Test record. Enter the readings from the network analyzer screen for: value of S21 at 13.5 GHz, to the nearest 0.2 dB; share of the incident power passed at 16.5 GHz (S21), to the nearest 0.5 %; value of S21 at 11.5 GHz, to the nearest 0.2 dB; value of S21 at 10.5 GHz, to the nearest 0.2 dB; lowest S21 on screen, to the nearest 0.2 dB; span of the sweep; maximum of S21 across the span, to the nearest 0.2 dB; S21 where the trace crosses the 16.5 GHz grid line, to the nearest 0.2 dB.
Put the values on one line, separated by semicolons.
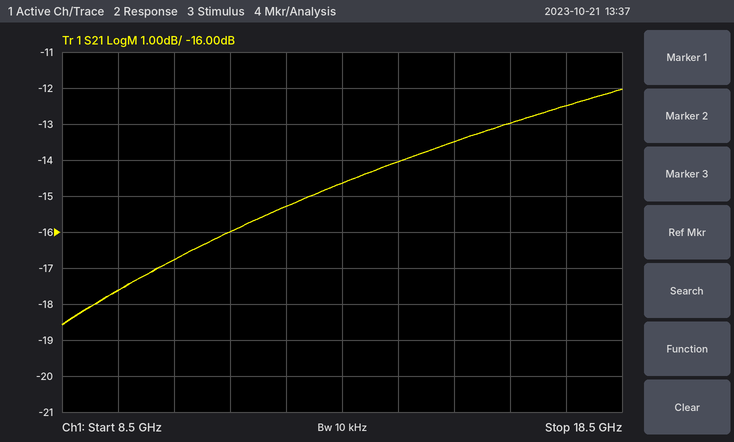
-14.6 dB; 5.0 %; -16.0 dB; -16.8 dB; -18.6 dB; 10 GHz; -12.0 dB; -13.0 dB
